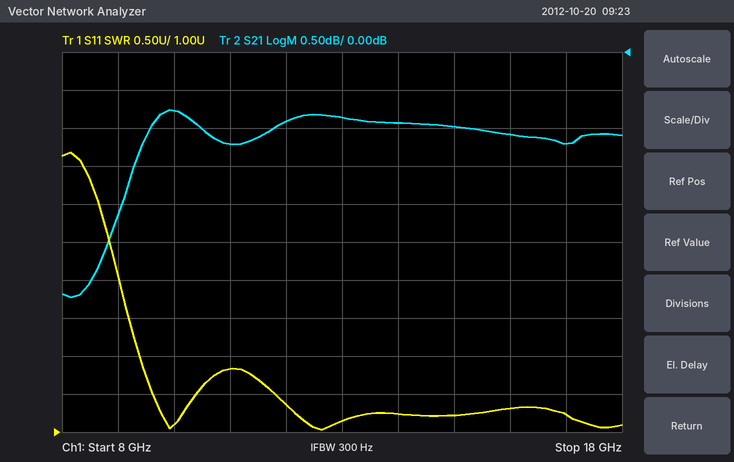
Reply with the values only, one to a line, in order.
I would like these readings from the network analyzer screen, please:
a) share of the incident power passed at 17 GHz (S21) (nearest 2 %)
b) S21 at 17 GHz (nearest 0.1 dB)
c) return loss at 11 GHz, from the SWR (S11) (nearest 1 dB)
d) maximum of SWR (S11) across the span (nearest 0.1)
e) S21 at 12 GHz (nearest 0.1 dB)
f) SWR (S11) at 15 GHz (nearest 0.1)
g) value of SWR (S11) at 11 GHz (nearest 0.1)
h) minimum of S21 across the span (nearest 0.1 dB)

76 %
-1.2 dB
11 dB
4.7
-0.9 dB
1.2
1.8
-3.2 dB
